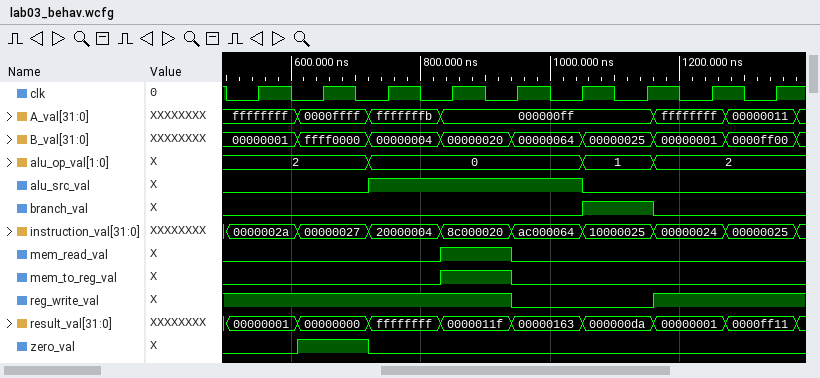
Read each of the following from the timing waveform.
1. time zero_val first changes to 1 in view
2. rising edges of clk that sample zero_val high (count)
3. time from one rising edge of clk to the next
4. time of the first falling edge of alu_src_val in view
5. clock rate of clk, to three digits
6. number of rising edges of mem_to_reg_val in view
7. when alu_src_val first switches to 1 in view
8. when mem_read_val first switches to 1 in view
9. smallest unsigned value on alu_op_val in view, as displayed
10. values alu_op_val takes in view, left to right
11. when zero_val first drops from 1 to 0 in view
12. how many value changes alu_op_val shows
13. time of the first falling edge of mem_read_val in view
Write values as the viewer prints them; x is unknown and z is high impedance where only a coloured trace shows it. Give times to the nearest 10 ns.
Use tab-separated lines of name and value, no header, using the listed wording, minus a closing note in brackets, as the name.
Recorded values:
time zero_val first changes to 1 in view	610 ns
rising edges of clk that sample zero_val high	1
time from one rising edge of clk to the next	100 ns
time of the first falling edge of alu_src_val in view	1050 ns
clock rate of clk, to three digits	10.0 MHz
number of rising edges of mem_to_reg_val in view	1
when alu_src_val first switches to 1 in view	720 ns
when mem_read_val first switches to 1 in view	830 ns
smallest unsigned value on alu_op_val in view, as displayed	0
values alu_op_val takes in view, left to right	2, 0, 1, 2
when zero_val first drops from 1 to 0 in view	720 ns
how many value changes alu_op_val shows	3
time of the first falling edge of mem_read_val in view	940 ns
